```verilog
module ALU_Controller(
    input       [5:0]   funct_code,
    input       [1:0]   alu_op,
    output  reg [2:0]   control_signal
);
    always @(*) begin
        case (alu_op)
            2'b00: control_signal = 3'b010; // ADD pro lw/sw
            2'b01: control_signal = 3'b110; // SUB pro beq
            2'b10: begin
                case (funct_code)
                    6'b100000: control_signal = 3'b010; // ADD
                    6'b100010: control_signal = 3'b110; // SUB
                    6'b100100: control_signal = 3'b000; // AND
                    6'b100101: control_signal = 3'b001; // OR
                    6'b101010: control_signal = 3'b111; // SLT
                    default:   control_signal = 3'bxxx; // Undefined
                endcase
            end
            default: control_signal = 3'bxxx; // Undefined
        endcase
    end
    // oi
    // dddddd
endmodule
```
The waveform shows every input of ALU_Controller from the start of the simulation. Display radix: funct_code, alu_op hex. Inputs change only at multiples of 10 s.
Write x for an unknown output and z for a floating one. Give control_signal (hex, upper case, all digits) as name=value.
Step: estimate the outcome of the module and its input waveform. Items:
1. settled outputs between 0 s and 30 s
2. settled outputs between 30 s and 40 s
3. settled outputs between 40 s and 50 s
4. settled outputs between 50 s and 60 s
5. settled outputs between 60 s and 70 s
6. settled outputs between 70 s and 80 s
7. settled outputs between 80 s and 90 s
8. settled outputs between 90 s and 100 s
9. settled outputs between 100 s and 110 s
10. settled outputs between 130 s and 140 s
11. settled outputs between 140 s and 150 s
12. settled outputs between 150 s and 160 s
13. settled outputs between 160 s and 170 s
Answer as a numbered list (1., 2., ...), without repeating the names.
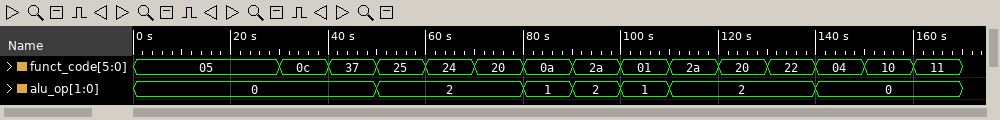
1. control_signal=2
2. control_signal=2
3. control_signal=2
4. control_signal=1
5. control_signal=0
6. control_signal=2
7. control_signal=6
8. control_signal=7
9. control_signal=6
10. control_signal=6
11. control_signal=2
12. control_signal=2
13. control_signal=2
